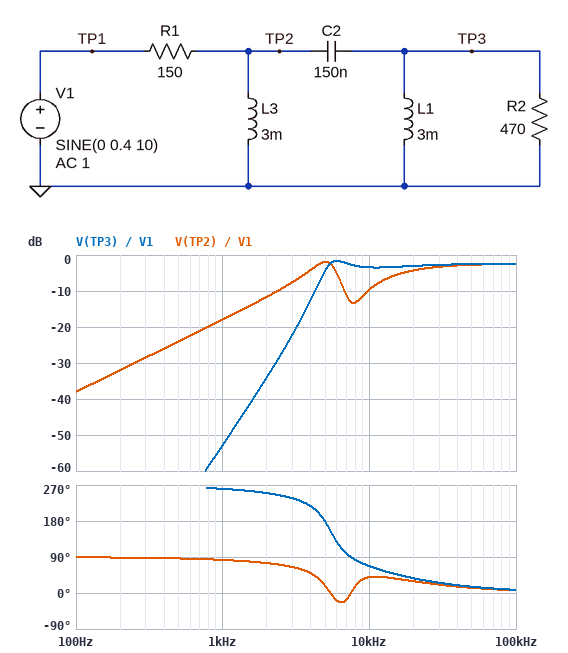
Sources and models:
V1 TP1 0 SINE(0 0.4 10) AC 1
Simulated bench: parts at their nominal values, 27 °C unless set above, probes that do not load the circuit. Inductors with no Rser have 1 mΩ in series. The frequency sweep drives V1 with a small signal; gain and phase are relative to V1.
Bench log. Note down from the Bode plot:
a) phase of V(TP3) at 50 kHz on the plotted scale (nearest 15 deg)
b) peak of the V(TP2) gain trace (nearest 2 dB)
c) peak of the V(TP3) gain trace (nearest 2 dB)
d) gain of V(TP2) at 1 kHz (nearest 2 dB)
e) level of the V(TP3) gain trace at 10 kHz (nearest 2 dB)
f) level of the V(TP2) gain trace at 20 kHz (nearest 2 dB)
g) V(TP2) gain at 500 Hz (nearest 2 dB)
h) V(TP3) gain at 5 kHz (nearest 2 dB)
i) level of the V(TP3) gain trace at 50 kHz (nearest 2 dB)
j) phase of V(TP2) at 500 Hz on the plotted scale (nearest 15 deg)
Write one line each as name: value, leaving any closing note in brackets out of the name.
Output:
phase of V(TP3) at 50 kHz on the plotted scale: 15 deg
peak of the V(TP2) gain trace: -2 dB
peak of the V(TP3) gain trace: -2 dB
gain of V(TP2) at 1 kHz: -18 dB
level of the V(TP3) gain trace at 10 kHz: -4 dB
level of the V(TP2) gain trace at 20 kHz: -4 dB
V(TP2) gain at 500 Hz: -24 dB
V(TP3) gain at 5 kHz: -4 dB
level of the V(TP3) gain trace at 50 kHz: -2 dB
phase of V(TP2) at 500 Hz on the plotted scale: 90 deg
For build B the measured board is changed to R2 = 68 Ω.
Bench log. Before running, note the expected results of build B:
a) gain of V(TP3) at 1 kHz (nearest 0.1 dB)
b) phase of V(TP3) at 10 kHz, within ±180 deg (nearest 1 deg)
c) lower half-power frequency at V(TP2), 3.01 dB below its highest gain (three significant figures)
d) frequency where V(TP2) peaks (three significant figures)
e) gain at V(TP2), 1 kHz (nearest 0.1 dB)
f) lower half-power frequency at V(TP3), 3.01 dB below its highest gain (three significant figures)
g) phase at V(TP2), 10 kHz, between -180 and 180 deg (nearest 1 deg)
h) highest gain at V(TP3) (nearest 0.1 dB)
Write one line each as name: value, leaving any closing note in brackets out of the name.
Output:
gain of V(TP3) at 1 kHz: -53.1 dB
phase of V(TP3) at 10 kHz, within ±180 deg: 63 deg
lower half-power frequency at V(TP2), 3.01 dB below its highest gain: 3.64 kHz
frequency where V(TP2) peaks: 5.87 kHz
gain at V(TP2), 1 kHz: -17.9 dB
lower half-power frequency at V(TP3), 3.01 dB below its highest gain: 5.34 kHz
phase at V(TP2), 10 kHz, between -180 and 180 deg: -12 deg
highest gain at V(TP3): -9.7 dB
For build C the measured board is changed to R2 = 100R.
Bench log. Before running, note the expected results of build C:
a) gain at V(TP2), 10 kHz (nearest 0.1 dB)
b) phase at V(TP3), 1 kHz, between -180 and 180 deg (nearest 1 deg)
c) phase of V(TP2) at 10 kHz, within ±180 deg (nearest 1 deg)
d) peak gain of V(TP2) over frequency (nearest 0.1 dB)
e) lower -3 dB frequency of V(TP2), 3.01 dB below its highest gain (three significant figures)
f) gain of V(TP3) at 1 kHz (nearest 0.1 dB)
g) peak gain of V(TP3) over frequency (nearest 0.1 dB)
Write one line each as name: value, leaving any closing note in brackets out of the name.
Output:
gain at V(TP2), 10 kHz: -6.6 dB
phase at V(TP3), 1 kHz, between -180 and 180 deg: -108 deg
phase of V(TP2) at 10 kHz, within ±180 deg: -4 deg
peak gain of V(TP2) over frequency: -3.1 dB
lower -3 dB frequency of V(TP2), 3.01 dB below its highest gain: 3.47 kHz
gain of V(TP3) at 1 kHz: -52.9 dB
peak gain of V(TP3) over frequency: -7.8 dB
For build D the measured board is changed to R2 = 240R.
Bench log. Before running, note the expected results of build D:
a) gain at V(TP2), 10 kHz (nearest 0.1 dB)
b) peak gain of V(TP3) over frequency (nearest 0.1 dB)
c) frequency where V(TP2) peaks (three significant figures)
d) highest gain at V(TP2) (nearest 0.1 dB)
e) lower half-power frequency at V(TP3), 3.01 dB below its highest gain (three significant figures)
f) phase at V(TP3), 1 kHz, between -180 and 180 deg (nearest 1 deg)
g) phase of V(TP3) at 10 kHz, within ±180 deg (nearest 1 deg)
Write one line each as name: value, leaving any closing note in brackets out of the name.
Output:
gain at V(TP2), 10 kHz: -8.9 dB
peak gain of V(TP3) over frequency: -4.0 dB
frequency where V(TP2) peaks: 4.97 kHz
highest gain at V(TP2): -2.7 dB
lower half-power frequency at V(TP3), 3.01 dB below its highest gain: 4.87 kHz
phase at V(TP3), 1 kHz, between -180 and 180 deg: -102 deg
phase of V(TP3) at 10 kHz, within ±180 deg: 66 deg
